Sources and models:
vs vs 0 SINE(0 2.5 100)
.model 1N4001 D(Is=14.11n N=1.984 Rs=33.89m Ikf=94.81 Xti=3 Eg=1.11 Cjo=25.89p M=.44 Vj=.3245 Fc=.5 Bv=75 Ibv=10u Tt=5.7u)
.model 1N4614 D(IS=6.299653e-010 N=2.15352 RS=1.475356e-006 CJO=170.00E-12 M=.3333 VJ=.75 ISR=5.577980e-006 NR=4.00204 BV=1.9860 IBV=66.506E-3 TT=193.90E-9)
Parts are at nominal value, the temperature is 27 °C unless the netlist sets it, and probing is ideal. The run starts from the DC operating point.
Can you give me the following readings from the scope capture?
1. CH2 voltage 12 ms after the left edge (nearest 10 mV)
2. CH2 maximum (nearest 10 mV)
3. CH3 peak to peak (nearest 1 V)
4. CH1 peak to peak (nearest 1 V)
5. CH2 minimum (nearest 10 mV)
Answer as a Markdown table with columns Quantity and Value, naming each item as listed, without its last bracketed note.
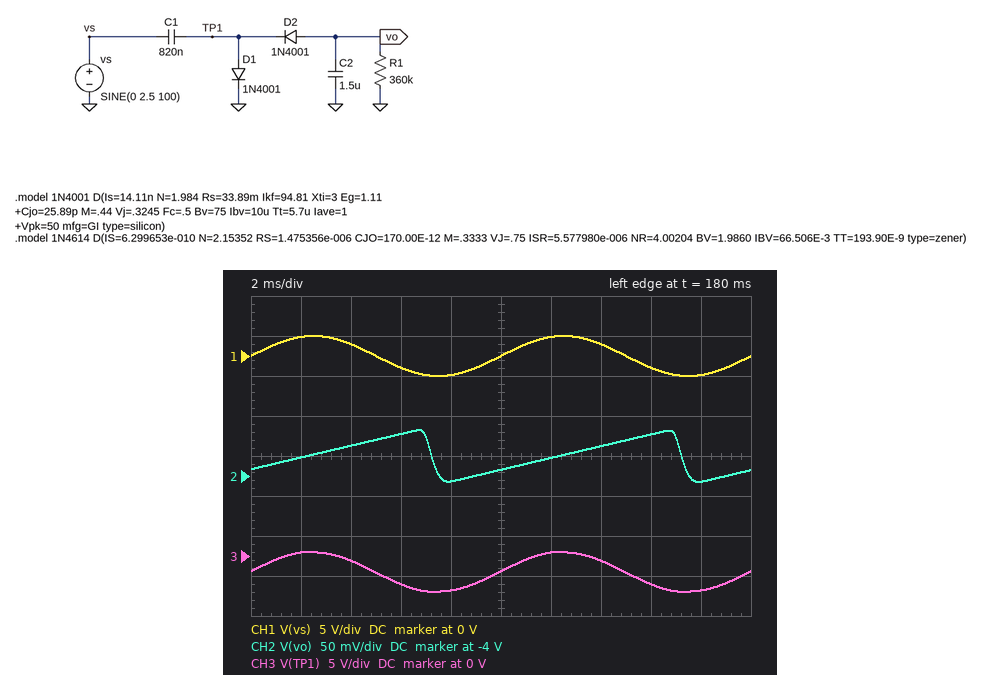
| Quantity | Value |
|---|---|
| CH2 voltage 12 ms after the left edge | -3.98 V |
| CH2 maximum | -3.94 V |
| CH3 peak to peak | 5 V |
| CH1 peak to peak | 5 V |
| CH2 minimum | -4.01 V |
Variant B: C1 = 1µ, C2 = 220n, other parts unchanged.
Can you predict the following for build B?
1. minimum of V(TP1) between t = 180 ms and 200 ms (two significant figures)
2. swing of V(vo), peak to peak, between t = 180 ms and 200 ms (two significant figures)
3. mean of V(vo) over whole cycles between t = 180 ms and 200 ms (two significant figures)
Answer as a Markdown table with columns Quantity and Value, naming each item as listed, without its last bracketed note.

| Quantity | Value |
|---|---|
| minimum of V(TP1) between t = 180 ms and 200 ms | -4.5 V |
| swing of V(vo), peak to peak, between t = 180 ms and 200 ms | 410 mV |
| mean of V(vo) over whole cycles between t = 180 ms and 200 ms | -3.9 V |
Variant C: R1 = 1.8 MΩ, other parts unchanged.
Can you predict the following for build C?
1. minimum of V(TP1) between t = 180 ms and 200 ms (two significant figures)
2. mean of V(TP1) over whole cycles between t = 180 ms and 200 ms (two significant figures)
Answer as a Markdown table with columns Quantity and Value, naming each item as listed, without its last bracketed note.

| Quantity | Value |
|---|---|
| minimum of V(TP1) between t = 180 ms and 200 ms | -4.6 V |
| mean of V(TP1) over whole cycles between t = 180 ms and 200 ms | -2.1 V |
